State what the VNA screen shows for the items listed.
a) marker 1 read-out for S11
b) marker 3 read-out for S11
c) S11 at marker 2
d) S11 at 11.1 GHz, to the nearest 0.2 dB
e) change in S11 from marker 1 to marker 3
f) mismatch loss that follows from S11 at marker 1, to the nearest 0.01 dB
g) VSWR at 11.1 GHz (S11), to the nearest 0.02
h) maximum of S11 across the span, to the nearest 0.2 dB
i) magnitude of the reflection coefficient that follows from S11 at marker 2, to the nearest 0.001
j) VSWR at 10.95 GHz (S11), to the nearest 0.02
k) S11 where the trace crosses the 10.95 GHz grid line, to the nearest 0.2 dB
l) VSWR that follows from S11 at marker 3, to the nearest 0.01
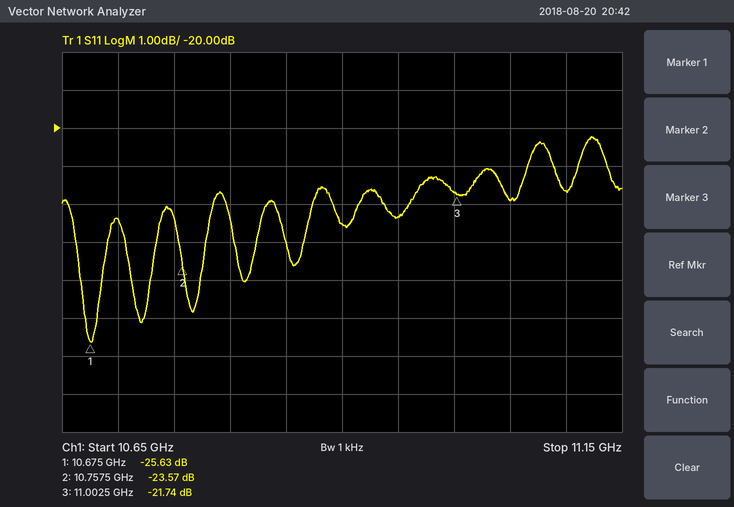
-25.63 dB
-21.74 dB
-23.57 dB
-21.6 dB
3.89 dB
0.01 dB
1.18
-20.2 dB
0.066
1.16
-22.4 dB
1.18
